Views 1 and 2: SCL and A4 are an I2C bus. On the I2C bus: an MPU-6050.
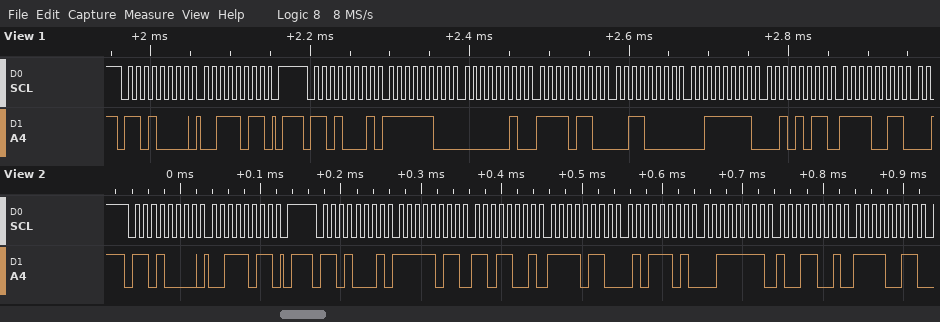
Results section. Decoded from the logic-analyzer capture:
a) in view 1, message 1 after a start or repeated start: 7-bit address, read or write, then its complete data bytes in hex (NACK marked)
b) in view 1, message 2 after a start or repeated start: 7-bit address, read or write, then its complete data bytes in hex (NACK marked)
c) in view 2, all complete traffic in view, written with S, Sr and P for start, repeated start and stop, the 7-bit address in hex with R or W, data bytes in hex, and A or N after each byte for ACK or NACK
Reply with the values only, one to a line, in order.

0x68 write: 3B
0x68 read: FC 02 F6 30 3F 2B F3
S 68W A 3B A P S 68R A FB A D9 A F6 A 5D A 3F A 99 A F3 A
